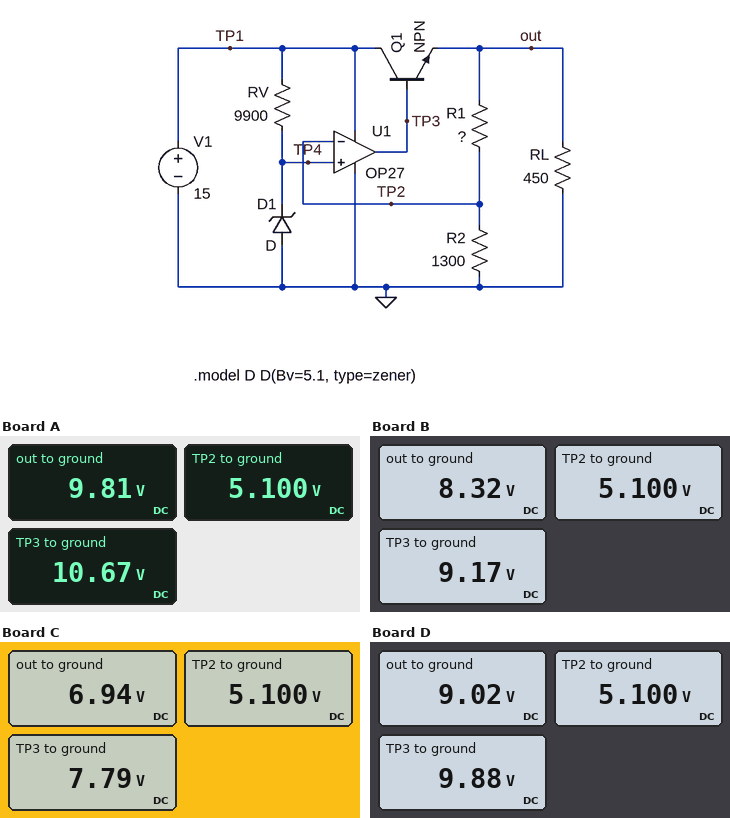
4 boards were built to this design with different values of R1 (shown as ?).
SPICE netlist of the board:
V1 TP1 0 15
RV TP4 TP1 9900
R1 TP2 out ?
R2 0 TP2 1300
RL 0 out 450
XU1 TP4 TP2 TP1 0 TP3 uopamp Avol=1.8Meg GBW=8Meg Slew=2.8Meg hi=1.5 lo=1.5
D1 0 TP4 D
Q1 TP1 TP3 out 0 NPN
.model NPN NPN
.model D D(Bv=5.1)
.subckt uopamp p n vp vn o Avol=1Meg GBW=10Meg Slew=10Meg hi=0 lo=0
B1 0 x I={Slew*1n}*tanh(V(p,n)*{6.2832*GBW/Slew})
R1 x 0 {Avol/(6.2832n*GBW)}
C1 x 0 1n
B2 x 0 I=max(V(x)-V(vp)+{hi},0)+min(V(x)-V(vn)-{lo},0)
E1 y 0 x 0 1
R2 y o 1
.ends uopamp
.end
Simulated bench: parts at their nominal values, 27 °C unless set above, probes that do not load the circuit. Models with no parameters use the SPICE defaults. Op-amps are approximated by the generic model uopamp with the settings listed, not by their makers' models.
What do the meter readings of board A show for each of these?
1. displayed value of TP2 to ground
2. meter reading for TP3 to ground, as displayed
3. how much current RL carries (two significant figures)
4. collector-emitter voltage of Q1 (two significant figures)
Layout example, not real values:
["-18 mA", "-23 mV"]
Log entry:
["5.100 V", "10.67 V", "22 mA", "5.2 V"]
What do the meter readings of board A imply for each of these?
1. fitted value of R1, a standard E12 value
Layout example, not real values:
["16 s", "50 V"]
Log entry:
["1.2 kΩ"]
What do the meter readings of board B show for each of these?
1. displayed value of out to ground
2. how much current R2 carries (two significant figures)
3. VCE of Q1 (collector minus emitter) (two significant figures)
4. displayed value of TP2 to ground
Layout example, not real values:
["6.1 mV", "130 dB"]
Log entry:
["8.32 V", "3.9 mA", "6.7 V", "5.100 V"]
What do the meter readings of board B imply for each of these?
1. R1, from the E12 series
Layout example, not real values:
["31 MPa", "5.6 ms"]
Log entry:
["820 Ω"]
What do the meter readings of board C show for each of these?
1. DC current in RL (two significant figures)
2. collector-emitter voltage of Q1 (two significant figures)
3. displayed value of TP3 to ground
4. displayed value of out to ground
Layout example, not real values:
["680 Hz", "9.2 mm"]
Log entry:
["15 mA", "8.1 V", "7.79 V", "6.94 V"]
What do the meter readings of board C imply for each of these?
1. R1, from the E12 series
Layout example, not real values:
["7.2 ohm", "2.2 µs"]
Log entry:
["470 Ω"]
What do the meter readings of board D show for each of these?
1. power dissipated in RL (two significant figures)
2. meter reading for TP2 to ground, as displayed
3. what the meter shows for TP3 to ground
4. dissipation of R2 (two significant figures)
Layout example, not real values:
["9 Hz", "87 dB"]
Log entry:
["180 mW", "5.100 V", "9.88 V", "20 mW"]
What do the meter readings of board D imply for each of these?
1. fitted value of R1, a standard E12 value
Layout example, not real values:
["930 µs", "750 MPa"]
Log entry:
["1 kΩ"]
